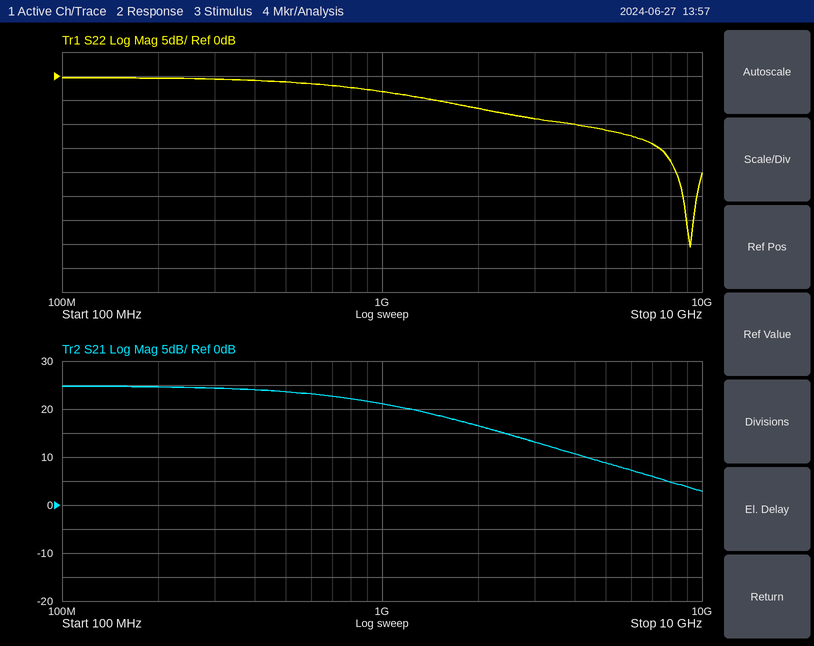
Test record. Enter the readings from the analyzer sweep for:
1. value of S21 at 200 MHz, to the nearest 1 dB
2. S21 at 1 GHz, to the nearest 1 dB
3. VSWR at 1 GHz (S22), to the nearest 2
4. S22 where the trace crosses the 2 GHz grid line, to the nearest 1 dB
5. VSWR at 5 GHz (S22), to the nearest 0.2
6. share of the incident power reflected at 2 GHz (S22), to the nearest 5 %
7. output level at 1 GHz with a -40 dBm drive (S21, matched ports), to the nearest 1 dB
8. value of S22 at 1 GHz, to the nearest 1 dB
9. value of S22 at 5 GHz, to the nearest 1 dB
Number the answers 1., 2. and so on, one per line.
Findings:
1. 25 dB
2. 21 dB
3. 6
4. -7 dB
5. 1.8
6. 20 %
7. -19 dBm
8. -3 dB
9. -11 dB
